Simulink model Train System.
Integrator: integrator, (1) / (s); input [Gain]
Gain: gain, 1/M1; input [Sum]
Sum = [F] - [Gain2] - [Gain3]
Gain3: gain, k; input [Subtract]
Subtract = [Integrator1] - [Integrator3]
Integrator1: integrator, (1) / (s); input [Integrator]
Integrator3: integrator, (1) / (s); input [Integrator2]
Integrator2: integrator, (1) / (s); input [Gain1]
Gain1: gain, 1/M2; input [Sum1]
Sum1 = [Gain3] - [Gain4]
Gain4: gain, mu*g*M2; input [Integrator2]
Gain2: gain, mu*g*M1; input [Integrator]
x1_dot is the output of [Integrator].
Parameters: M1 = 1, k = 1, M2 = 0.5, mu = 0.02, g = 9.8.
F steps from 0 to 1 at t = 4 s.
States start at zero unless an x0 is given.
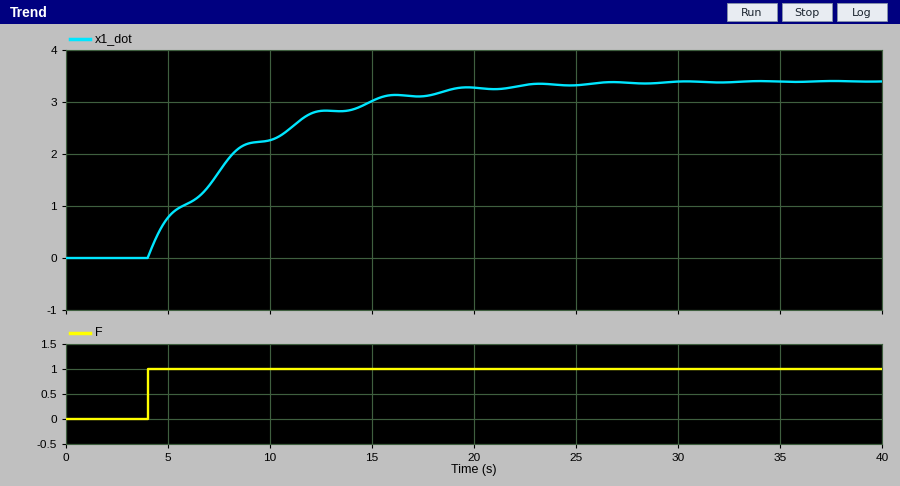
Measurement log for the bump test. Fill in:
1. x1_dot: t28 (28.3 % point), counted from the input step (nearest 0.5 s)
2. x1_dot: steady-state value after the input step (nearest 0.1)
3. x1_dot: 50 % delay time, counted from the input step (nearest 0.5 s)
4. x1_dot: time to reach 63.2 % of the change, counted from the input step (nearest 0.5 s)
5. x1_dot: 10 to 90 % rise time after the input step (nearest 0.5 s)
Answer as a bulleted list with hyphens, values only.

- 1.5 s
- 3.4
- 3.5 s
- 4.5 s
- 11.0 s
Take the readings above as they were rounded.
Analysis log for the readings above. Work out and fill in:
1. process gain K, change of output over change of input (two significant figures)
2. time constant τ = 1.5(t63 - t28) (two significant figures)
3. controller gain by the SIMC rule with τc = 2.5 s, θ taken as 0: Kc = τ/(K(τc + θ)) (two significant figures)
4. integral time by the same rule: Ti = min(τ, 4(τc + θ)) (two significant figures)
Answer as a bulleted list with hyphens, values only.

- 3.4
- 4.5 s
- 0.53
- 4.5 s
